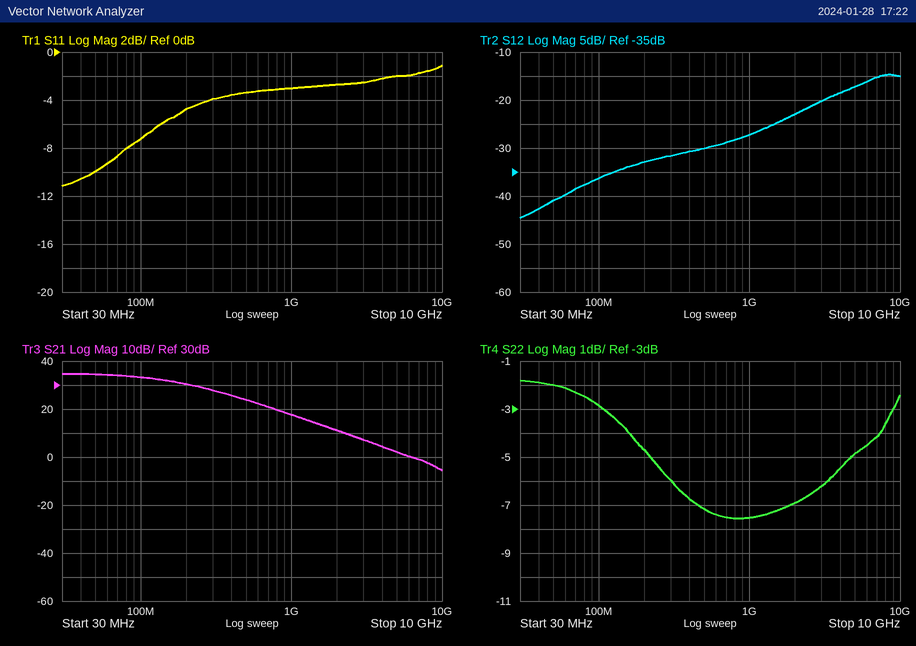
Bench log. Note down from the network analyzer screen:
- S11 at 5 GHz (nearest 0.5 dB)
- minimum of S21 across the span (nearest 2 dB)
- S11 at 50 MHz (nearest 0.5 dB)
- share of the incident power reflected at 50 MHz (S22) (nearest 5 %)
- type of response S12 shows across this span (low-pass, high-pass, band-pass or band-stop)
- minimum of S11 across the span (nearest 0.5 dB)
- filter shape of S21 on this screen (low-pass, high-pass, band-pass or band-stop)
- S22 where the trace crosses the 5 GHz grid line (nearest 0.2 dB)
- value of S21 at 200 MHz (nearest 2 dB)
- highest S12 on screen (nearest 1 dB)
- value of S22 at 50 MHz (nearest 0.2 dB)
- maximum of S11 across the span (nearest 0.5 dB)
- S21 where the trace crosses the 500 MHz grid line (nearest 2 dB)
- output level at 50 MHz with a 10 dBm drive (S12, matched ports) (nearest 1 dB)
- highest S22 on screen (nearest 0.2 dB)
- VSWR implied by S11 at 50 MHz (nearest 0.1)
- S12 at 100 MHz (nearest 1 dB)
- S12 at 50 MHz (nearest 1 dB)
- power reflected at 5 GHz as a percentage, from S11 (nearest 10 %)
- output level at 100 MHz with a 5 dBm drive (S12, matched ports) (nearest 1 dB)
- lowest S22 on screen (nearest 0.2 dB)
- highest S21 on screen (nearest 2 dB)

-2.0 dB
-6 dB
-10.0 dB
65 %
high-pass
-11.0 dB
low-pass
-4.8 dB
30 dB
-15 dB
-2.0 dB
-1.0 dB
24 dB
-31 dBm
-1.8 dB
1.9
-36 dB
-41 dB
60 %
-31 dBm
-7.6 dB
34 dB
